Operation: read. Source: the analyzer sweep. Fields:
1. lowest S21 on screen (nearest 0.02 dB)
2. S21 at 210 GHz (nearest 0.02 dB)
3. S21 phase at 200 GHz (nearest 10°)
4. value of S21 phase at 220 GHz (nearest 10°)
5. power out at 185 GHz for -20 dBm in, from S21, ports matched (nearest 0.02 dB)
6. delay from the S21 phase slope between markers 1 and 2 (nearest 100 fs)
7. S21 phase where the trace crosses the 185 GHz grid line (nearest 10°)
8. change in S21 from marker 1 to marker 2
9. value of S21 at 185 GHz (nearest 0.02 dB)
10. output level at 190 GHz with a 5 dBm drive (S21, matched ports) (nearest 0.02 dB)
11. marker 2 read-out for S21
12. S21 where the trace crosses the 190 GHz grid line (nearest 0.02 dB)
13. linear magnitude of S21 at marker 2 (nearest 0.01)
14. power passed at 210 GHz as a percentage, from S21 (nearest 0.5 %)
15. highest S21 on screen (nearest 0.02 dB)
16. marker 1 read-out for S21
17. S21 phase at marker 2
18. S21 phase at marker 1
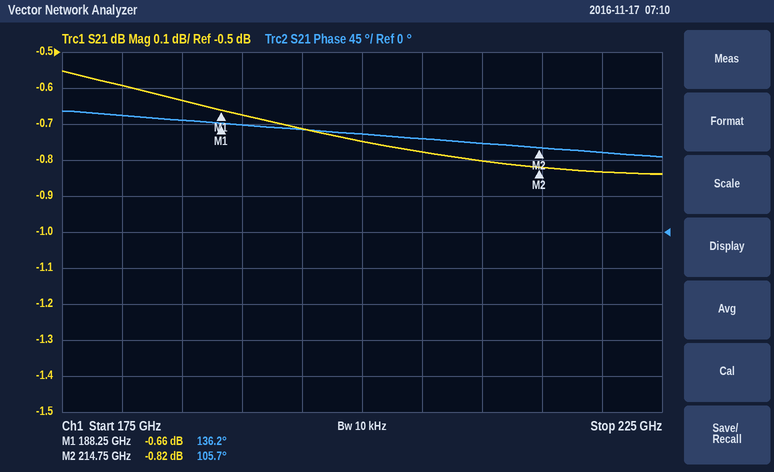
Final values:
-0.84 dB
-0.80 dB
120°
100°
-20.64 dBm
3.2 ps
140°
-0.16 dB
-0.64 dB
4.32 dBm
-0.82 dB
-0.68 dB
0.91
83.0 %
-0.56 dB
-0.66 dB
105.7°
136.2°
